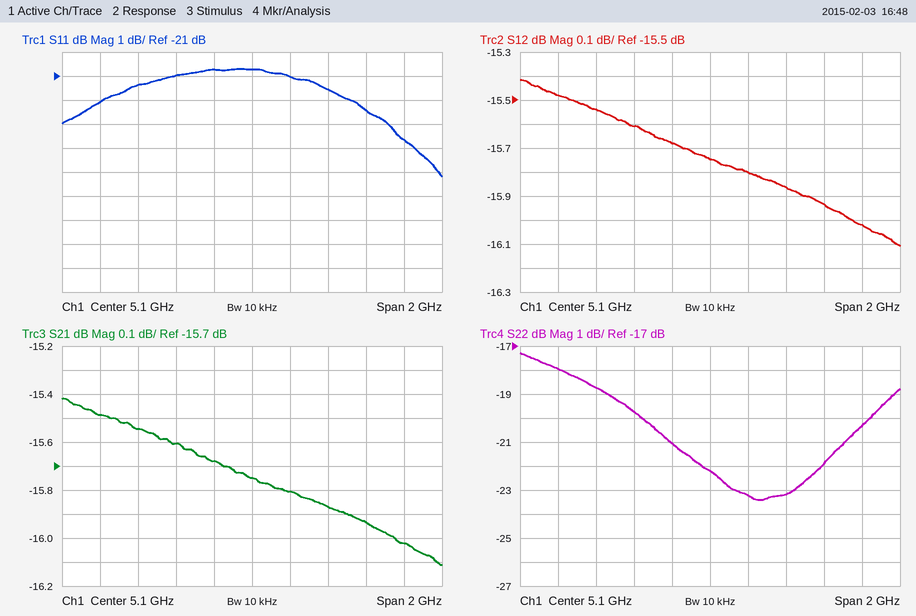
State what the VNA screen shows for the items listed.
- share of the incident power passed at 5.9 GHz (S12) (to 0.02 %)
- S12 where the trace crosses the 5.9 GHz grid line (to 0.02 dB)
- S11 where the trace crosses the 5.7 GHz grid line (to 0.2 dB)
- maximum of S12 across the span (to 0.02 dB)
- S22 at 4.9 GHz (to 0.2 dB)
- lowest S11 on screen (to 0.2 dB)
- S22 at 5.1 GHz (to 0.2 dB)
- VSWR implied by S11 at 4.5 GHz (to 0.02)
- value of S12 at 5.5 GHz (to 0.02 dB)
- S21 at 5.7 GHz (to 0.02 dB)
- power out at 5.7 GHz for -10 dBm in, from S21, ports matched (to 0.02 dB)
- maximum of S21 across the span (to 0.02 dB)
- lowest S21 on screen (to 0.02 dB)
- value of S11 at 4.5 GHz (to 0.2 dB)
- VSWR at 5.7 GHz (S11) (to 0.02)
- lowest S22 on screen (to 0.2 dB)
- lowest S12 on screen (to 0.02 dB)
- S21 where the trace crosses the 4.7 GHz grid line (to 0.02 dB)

2.50 %
-16.02 dB
-22.4 dB
-15.42 dB
-21.0 dB
-25.2 dB
-22.2 dB
1.18
-15.86 dB
-15.94 dB
-25.94 dBm
-15.42 dB
-16.12 dB
-21.4 dB
1.16
-23.4 dB
-16.10 dB
-15.60 dB
